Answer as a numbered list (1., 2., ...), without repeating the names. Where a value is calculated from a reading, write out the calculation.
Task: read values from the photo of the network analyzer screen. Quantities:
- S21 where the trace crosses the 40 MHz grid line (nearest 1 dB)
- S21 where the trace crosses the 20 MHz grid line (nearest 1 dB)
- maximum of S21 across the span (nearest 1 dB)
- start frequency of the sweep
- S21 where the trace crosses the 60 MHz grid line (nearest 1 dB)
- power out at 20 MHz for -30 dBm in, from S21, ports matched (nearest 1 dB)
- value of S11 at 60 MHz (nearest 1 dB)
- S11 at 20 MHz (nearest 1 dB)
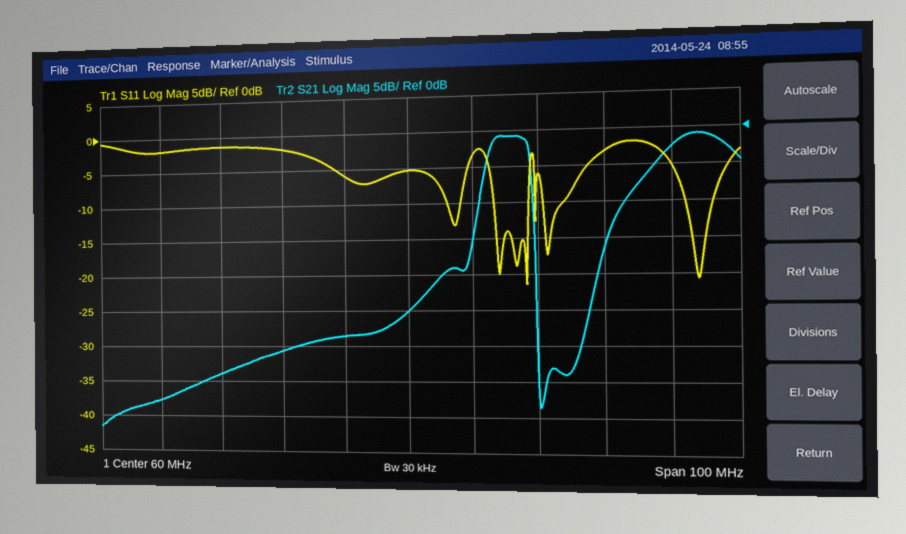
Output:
1. -31 dB
2. -38 dB
3. -1 dB
4. 10 MHz
5. -25 dB
6. -30 dBm + (-38 dB) = -68 dBm
7. -5 dB
8. -2 dB
